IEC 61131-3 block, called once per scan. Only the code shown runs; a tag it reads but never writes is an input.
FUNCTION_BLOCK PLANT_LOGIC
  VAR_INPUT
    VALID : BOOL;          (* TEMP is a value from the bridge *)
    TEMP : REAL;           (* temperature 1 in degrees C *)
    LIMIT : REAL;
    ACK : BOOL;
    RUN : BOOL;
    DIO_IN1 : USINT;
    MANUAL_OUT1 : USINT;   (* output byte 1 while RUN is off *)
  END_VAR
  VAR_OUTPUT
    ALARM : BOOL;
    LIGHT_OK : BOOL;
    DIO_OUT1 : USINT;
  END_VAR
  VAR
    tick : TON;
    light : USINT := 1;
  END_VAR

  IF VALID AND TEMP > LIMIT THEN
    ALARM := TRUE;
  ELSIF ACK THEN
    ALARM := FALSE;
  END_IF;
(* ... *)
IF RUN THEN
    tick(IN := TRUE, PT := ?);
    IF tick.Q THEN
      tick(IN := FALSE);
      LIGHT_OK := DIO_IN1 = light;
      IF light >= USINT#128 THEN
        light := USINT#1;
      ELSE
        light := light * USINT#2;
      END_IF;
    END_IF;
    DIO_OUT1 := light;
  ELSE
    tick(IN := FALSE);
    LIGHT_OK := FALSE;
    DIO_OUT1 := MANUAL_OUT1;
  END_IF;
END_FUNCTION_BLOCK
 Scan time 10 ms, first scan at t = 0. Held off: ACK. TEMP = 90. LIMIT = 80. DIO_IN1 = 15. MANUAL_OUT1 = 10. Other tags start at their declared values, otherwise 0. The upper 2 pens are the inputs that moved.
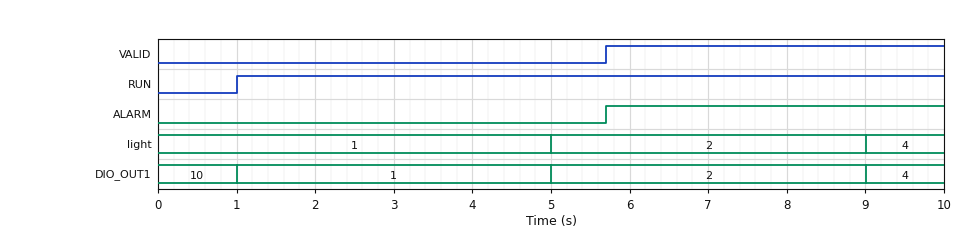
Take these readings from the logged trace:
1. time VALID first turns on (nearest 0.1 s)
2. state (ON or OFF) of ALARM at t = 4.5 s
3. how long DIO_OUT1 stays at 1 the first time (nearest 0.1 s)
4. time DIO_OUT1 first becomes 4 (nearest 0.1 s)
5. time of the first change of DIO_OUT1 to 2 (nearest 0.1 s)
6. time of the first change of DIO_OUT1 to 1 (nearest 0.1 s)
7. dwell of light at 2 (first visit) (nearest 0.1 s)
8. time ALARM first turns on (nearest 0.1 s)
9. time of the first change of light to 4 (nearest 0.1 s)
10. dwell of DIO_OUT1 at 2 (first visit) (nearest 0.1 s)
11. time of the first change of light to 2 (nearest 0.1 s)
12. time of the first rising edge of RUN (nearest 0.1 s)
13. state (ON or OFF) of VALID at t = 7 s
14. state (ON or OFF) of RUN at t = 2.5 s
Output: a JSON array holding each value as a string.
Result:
["5.7 s", "OFF", "4.0 s", "9.0 s", "5.0 s", "1.0 s", "4.0 s", "5.7 s", "9.0 s", "4.0 s", "5.0 s", "1.0 s", "ON", "ON"]
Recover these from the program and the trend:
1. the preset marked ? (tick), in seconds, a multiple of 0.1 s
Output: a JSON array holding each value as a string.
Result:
["4.0 s"]
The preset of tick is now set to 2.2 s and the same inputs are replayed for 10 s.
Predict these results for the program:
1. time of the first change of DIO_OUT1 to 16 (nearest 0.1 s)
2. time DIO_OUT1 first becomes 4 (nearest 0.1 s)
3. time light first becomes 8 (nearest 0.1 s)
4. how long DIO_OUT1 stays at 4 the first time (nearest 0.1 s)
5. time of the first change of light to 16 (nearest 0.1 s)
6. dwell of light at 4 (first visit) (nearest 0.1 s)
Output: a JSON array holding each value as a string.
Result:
["9.8 s", "5.4 s", "7.6 s", "2.2 s", "9.8 s", "2.2 s"]
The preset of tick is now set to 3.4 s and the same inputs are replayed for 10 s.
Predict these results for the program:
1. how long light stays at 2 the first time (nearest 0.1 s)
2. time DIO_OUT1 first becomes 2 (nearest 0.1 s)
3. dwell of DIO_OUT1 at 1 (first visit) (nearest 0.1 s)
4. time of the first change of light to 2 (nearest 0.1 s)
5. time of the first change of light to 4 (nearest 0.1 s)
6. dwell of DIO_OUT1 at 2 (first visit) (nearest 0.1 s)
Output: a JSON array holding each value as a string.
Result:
["3.4 s", "4.4 s", "3.4 s", "4.4 s", "7.8 s", "3.4 s"]
